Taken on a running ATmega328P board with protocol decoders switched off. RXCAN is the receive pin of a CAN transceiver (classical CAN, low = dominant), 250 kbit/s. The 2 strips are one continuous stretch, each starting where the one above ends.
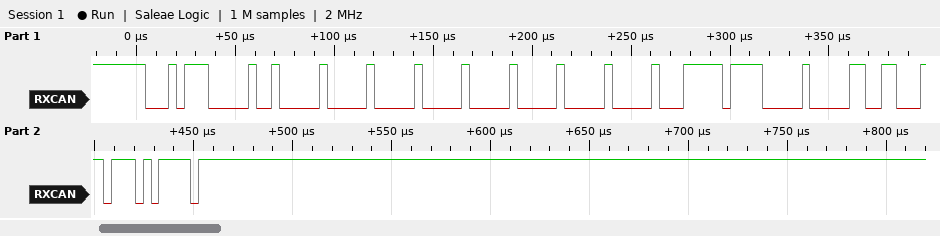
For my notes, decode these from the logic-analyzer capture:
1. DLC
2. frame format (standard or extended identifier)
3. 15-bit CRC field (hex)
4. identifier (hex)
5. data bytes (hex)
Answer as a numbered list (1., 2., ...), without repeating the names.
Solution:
1. 8
2. standard
3. 0x0DD7
4. 0x170
5. 00 00 00 00 00 FF 80 13
